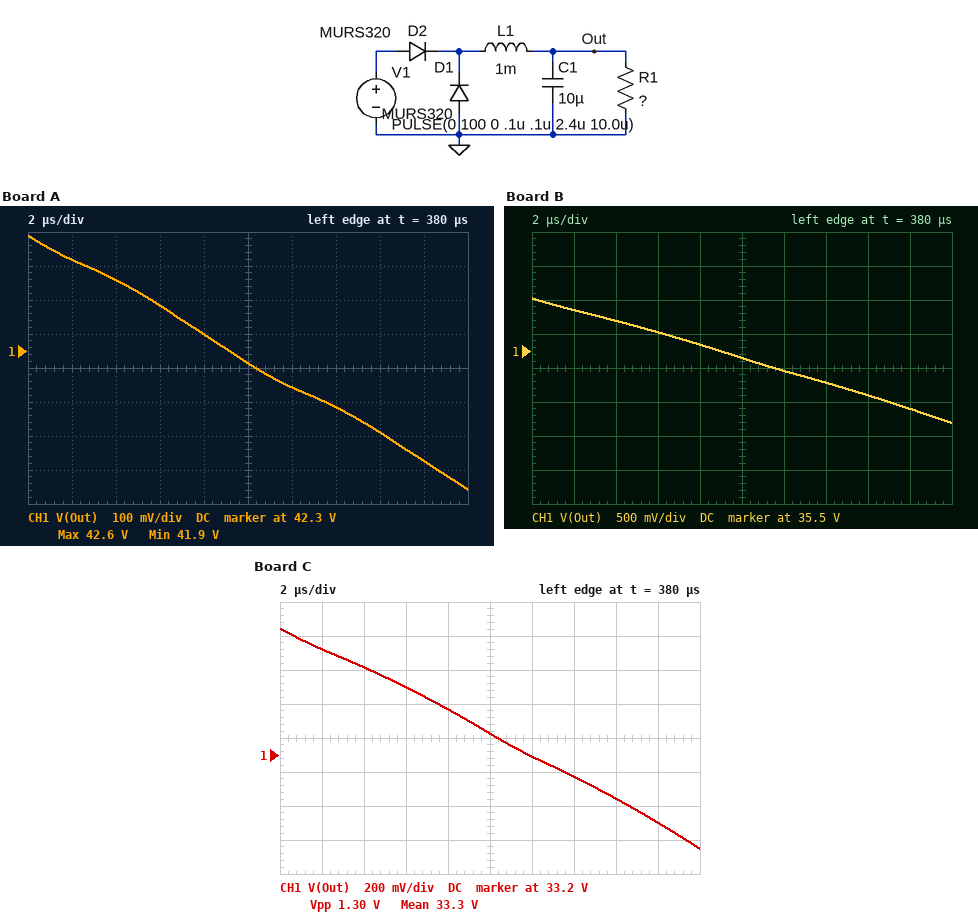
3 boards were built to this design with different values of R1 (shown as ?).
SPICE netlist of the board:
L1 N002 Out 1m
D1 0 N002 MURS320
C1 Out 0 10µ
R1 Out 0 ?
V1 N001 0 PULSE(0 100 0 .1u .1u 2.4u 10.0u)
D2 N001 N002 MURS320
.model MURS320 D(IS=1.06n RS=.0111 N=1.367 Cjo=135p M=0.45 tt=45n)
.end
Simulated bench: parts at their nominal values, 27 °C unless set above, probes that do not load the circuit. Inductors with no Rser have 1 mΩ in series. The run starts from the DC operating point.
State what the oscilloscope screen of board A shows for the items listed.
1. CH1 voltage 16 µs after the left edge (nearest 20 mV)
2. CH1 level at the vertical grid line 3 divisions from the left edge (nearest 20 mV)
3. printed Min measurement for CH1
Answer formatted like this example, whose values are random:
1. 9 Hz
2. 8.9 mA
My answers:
1. 42.06 V
2. 42.44 V
3. 41.9 V
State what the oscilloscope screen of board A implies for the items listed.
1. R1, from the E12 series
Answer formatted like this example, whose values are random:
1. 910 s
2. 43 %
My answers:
1. 100 Ω
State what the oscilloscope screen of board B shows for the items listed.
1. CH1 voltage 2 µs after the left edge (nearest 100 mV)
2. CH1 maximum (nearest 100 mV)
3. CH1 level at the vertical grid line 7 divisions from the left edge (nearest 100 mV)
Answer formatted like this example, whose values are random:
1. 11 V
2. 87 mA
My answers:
1. 36.1 V
2. 36.3 V
3. 35.0 V
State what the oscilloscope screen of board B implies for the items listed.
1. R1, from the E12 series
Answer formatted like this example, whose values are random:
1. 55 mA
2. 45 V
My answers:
1. 33 Ω
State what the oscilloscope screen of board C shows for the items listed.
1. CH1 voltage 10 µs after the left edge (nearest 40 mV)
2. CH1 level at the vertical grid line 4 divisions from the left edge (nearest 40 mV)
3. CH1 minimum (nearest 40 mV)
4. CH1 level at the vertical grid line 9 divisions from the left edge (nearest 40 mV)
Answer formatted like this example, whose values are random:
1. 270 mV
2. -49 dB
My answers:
1. 33.32 V
2. 33.48 V
3. 32.64 V
4. 32.80 V
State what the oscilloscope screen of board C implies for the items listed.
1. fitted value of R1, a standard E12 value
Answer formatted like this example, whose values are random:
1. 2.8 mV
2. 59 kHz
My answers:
1. 22 Ω
